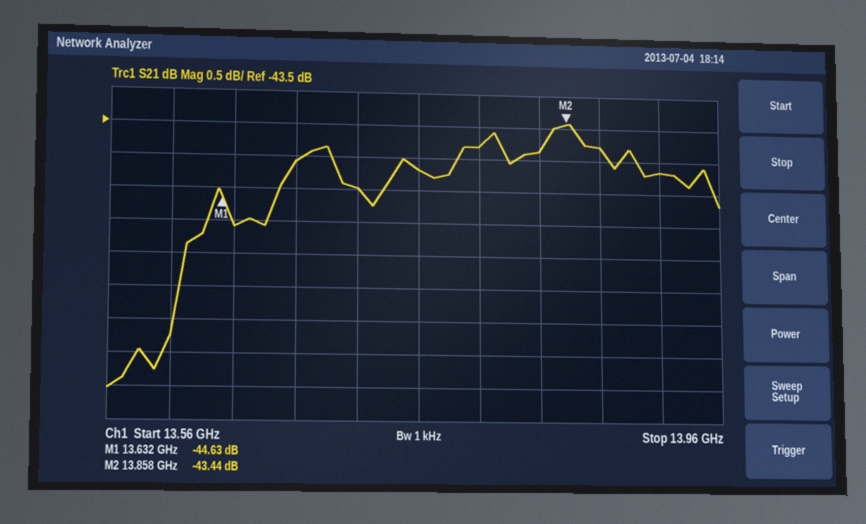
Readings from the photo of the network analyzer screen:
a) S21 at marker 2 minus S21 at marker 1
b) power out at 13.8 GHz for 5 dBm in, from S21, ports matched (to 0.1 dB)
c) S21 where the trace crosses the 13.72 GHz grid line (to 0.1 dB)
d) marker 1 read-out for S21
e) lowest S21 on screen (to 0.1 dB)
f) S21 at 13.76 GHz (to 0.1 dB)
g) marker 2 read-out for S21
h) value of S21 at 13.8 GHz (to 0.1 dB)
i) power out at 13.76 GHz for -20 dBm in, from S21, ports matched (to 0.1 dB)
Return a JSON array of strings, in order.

["1.19 dB", "-38.8 dBm", "-44.5 dB", "-44.63 dB", "-47.5 dB", "-44.2 dB", "-43.44 dB", "-43.8 dB", "-64.2 dBm"]
